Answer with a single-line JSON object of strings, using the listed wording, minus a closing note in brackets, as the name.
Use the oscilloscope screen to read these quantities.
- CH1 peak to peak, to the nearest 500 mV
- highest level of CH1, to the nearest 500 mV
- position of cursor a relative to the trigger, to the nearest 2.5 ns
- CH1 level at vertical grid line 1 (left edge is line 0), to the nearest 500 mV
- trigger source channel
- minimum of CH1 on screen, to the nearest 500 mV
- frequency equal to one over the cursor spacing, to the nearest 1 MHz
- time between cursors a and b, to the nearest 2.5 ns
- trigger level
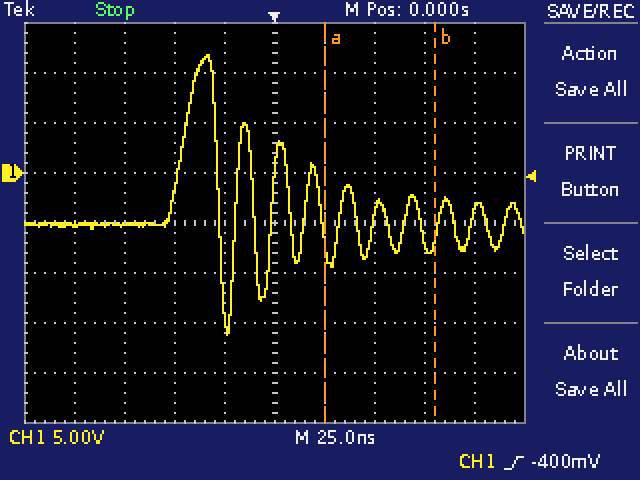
{"CH1 peak to peak, to the nearest 500 mV": "28.0 V", "highest level of CH1, to the nearest 500 mV": "12.0 V", "position of cursor a relative to the trigger, to the nearest 2.5 ns": "+25.0 ns", "CH1 level at vertical grid line 1 (left edge is line 0), to the nearest 500 mV": "-5.0 V", "trigger source channel": "CH1", "minimum of CH1 on screen, to the nearest 500 mV": "-16.0 V", "frequency equal to one over the cursor spacing, to the nearest 1 MHz": "18 MHz", "time between cursors a and b, to the nearest 2.5 ns": "55.0 ns", "trigger level": "-400 mV"}
